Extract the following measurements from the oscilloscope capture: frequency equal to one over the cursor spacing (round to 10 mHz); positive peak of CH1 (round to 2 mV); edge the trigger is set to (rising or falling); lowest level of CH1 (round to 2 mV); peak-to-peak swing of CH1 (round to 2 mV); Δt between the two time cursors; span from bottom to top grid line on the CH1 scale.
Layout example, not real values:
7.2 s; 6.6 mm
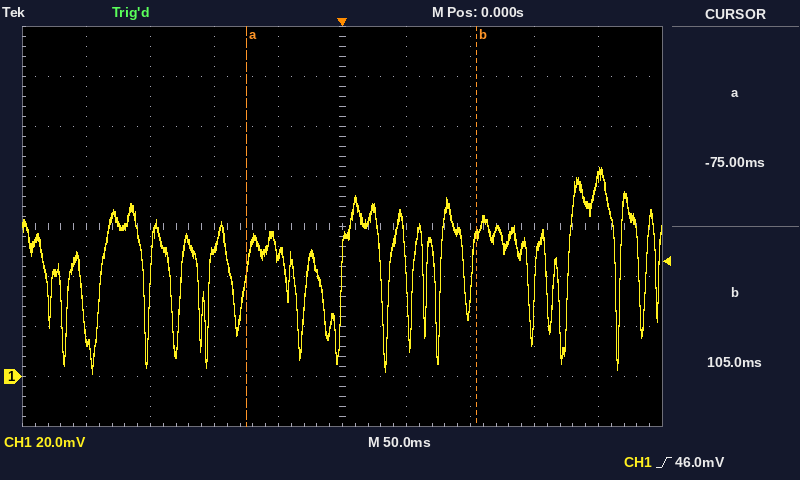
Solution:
5.56 Hz; 84 mV; rising; 2 mV; 82 mV; 180 ms; 160 mV
